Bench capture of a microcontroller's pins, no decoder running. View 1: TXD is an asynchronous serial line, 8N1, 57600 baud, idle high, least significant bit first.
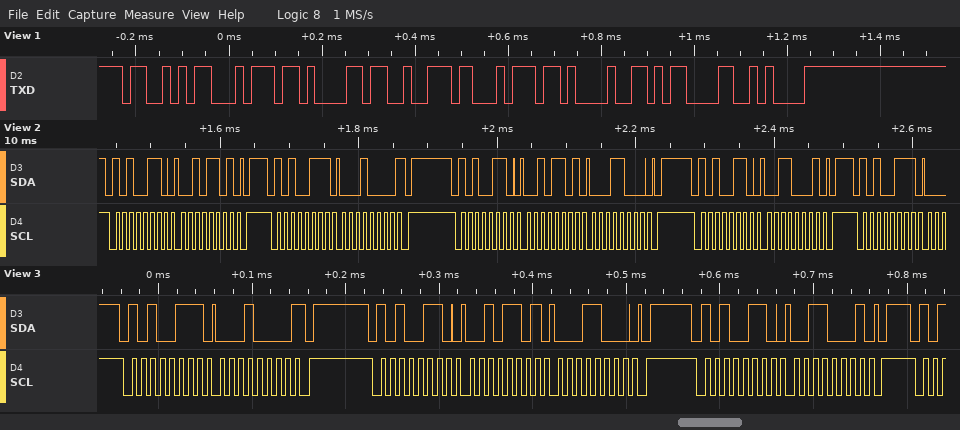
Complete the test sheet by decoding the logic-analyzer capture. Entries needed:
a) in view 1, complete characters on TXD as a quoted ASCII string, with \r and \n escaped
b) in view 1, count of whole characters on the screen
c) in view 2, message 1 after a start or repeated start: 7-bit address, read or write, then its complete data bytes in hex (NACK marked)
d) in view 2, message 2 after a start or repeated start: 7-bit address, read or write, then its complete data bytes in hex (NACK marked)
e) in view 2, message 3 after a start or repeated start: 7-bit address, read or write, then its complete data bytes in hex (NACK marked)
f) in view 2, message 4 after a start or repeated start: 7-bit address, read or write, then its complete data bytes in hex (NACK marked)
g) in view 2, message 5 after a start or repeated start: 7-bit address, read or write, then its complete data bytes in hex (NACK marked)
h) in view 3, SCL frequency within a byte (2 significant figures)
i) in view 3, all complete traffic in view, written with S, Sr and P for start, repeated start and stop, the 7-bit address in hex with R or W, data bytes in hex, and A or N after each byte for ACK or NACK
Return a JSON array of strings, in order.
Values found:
["\"Start!\\r\\n\"", "8", "0x53 write: 2D", "0x53 read: 10 NACK", "0x53 write: 2D 18", "0x53 write: 31", "0x53 read", "100 kHz", "S 53R A 10 N P S 53W A 2D A 18 A P S 53W A 31 A P"]
